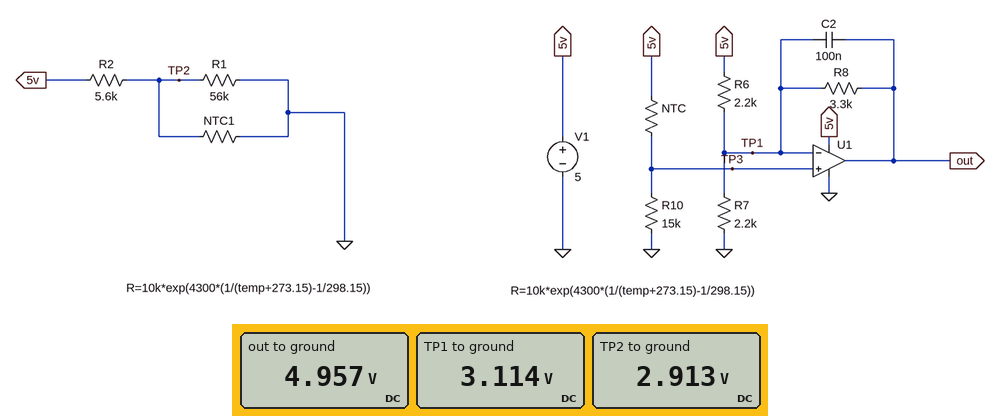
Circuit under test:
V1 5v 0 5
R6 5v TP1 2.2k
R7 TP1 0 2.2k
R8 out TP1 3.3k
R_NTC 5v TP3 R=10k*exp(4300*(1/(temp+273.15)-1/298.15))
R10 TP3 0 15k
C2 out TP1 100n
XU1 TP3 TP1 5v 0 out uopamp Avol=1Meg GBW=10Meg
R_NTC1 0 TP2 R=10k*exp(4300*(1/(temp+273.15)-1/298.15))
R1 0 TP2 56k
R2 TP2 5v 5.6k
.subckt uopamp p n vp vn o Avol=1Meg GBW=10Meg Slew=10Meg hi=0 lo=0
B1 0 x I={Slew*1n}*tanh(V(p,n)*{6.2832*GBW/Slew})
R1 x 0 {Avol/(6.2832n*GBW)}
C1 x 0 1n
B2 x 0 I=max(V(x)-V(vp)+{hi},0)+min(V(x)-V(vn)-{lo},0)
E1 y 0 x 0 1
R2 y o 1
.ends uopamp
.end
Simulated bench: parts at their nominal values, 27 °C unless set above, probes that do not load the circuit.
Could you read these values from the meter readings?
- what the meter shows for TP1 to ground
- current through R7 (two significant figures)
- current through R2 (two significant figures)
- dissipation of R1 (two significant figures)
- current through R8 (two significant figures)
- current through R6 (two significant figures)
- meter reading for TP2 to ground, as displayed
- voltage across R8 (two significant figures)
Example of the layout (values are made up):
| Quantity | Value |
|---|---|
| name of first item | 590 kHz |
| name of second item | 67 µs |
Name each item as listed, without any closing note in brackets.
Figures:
| Quantity | Value |
|---|---|
| what the meter shows for TP1 to ground | 3.114 V |
| current through R7 | 1.4 mA |
| current through R2 | 370 µA |
| dissipation of R1 | 150 µW |
| current through R8 | 560 µA |
| current through R6 | 860 µA |
| meter reading for TP2 to ground, as displayed | 2.913 V |
| voltage across R8 | 1.8 V |
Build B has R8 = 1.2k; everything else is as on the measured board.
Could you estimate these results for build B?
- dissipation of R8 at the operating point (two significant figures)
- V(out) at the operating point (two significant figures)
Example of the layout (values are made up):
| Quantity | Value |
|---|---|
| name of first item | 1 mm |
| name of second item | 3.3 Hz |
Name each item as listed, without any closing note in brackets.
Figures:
| Quantity | Value |
|---|---|
| dissipation of R8 at the operating point | 370 µW |
| V(out) at the operating point | 3.8 V |
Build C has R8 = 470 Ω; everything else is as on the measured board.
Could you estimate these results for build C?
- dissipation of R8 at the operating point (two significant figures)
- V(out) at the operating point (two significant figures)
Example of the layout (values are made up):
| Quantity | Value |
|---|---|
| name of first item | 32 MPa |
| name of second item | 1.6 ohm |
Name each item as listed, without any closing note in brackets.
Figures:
| Quantity | Value |
|---|---|
| dissipation of R8 at the operating point | 150 µW |
| V(out) at the operating point | 3.4 V |
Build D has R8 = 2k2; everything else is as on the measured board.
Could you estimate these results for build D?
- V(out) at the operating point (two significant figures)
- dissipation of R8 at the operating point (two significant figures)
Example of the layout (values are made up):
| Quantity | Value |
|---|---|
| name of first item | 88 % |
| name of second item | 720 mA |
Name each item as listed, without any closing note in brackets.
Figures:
| Quantity | Value |
|---|---|
| V(out) at the operating point | 4.3 V |
| dissipation of R8 at the operating point | 690 µW |
